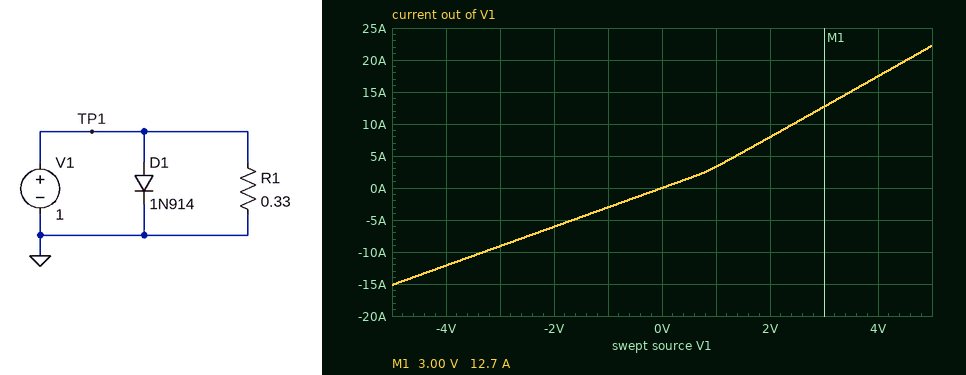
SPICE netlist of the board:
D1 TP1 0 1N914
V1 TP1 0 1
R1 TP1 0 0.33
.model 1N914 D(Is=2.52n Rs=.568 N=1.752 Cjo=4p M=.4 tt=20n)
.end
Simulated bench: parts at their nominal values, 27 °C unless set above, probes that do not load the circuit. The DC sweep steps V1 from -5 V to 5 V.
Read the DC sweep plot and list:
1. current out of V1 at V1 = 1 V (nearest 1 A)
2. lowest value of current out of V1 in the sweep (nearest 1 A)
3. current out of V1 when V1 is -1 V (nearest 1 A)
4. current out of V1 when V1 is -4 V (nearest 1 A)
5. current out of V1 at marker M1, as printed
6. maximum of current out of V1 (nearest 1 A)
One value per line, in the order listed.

3 A
-15 A
-3 A
-12 A
12.7 A
22 A
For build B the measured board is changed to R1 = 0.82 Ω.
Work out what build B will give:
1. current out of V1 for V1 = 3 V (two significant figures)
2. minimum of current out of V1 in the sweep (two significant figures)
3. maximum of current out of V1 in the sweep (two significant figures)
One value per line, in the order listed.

7.3 A
-6.1 A
13 A
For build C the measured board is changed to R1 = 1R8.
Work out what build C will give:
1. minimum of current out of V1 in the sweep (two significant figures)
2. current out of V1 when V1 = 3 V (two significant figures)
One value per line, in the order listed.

-2.8 A
5.3 A
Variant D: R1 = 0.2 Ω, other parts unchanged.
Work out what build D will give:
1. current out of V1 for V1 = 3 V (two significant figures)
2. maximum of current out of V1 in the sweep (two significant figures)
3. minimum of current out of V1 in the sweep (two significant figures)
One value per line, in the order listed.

19 A
32 A
-25 A
